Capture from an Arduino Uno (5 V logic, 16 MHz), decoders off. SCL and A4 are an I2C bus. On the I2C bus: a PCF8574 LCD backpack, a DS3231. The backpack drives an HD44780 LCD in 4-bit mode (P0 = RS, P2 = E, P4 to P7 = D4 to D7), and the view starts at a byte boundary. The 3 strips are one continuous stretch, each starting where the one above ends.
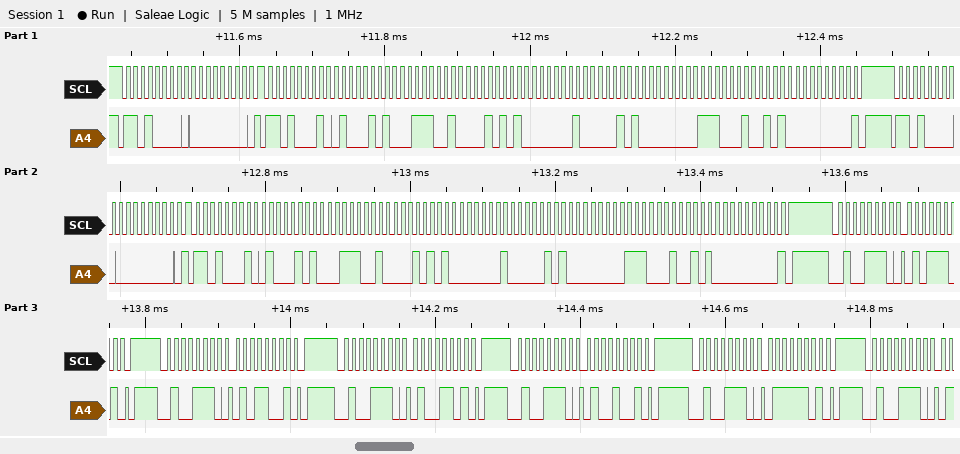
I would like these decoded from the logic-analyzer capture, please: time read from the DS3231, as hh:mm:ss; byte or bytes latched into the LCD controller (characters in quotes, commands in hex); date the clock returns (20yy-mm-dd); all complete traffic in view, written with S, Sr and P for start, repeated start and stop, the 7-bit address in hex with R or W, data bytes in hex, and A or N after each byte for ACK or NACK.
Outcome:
15:39:45
'T'
2025-07-14
S 68W A 00 A Sr 68R A 45 A 39 A 15 A 02 A 14 A 07 A 25 A 00 N P S 68W A 00 A Sr 68R A 45 A 39 A 15 A 02 A 14 A 07 A 25 A 00 N P S 27W A 5D A P S 27W A 59 A P S 27W A 4D A P S 27W A 49 A P S 27W A 7D A P S 27W A
